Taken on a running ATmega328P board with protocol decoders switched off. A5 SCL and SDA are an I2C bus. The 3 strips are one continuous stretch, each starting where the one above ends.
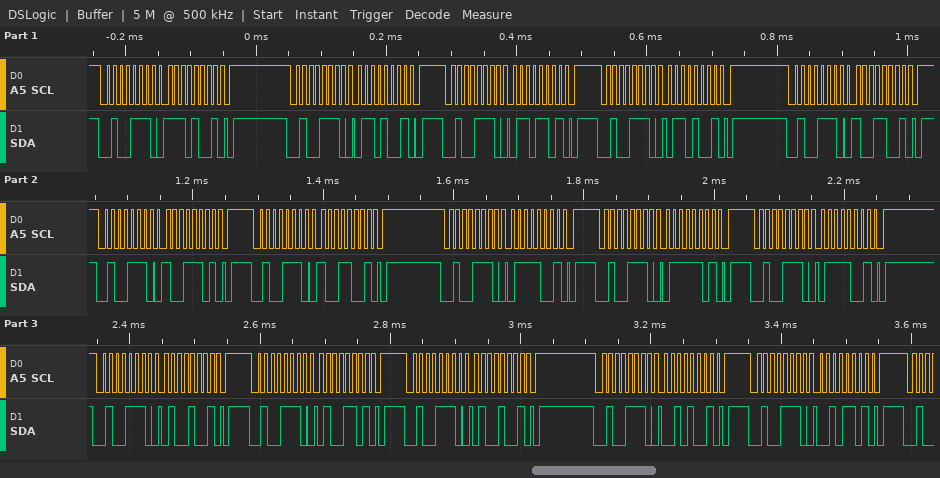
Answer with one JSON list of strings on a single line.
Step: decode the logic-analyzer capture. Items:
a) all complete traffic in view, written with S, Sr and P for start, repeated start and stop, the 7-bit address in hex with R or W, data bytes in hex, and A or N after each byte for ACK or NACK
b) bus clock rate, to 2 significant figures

["S 27W A E9 A P S 27W A 69 A P S 27W A 6D A P S 27W A 69 A P S 27W A 99 A P S 27W A 9D A P S 27W A 99 A P S 27W A 79 A P S 27W A 7D A P S 27W A 79 A P S 27W A 49 A P S 27W A 4D A P S 27W A 49 A P S 27W A 29 A P S 27W A 2D A P", "100 kHz"]
